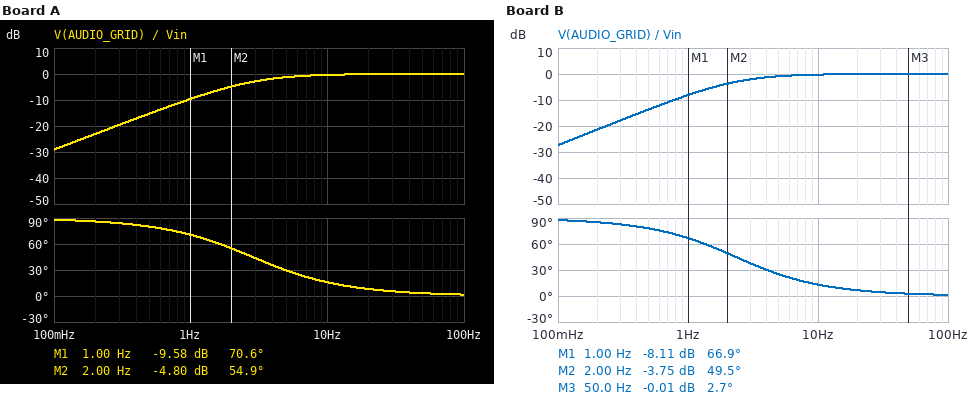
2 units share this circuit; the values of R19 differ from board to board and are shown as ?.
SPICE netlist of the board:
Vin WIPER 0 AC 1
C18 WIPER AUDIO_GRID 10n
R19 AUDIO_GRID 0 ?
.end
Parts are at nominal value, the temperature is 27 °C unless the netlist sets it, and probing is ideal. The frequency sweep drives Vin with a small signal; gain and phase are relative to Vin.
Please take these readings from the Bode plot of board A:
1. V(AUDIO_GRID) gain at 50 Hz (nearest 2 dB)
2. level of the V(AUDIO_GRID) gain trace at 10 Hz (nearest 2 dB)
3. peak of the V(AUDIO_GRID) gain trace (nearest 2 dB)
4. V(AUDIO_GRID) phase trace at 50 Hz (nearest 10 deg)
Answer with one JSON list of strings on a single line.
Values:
["0 dB", "0 dB", "0 dB", "0 deg"]
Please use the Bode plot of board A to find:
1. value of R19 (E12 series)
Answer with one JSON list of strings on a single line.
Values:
["5.6 MΩ"]
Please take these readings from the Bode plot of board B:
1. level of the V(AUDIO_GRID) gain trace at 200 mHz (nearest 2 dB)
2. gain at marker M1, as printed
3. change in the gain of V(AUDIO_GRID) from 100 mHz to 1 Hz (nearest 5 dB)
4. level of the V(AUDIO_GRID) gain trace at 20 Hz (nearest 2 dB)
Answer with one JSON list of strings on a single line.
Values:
["-22 dB", "-8.11 dB", "20 dB", "0 dB"]
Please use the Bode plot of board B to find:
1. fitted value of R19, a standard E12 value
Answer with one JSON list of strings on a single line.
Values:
["6.8 MΩ"]
